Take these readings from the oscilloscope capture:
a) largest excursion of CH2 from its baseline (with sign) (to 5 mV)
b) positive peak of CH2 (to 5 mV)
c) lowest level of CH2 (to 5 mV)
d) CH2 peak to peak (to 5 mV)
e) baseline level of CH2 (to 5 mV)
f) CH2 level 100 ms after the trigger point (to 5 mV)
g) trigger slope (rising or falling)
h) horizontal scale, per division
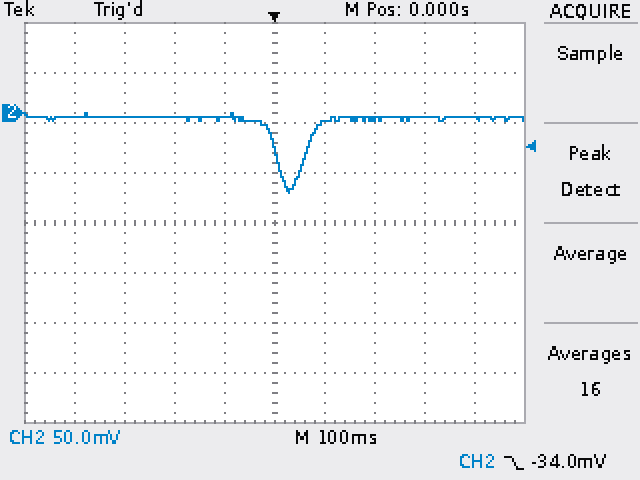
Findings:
-75 mV
0 mV
-80 mV
80 mV
-5 mV
-10 mV
falling
100 ms
